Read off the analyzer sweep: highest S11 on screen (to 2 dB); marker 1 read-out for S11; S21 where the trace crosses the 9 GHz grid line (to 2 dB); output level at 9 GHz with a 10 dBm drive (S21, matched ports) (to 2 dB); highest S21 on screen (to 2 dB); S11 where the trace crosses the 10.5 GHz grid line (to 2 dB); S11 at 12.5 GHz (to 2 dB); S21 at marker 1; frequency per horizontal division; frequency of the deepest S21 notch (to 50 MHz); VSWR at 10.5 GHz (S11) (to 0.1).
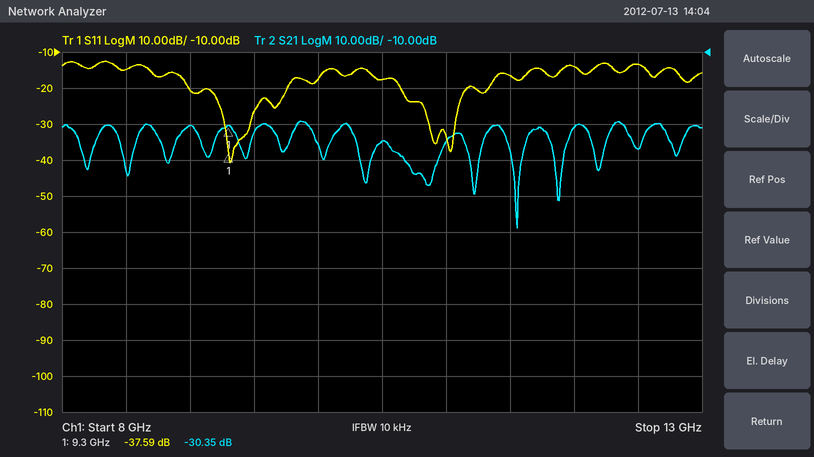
-12 dB
-37.59 dB
-30 dB
-20 dBm
-30 dB
-18 dB
-14 dB
-30.35 dB
500 MHz
11.55 GHz
1.3
